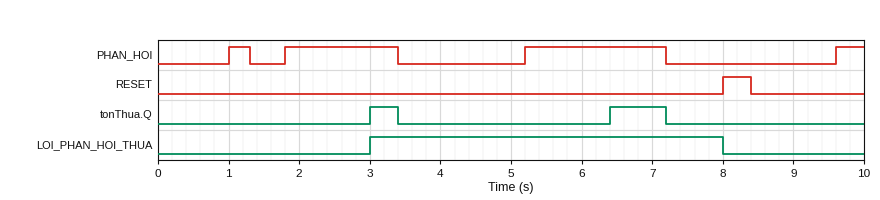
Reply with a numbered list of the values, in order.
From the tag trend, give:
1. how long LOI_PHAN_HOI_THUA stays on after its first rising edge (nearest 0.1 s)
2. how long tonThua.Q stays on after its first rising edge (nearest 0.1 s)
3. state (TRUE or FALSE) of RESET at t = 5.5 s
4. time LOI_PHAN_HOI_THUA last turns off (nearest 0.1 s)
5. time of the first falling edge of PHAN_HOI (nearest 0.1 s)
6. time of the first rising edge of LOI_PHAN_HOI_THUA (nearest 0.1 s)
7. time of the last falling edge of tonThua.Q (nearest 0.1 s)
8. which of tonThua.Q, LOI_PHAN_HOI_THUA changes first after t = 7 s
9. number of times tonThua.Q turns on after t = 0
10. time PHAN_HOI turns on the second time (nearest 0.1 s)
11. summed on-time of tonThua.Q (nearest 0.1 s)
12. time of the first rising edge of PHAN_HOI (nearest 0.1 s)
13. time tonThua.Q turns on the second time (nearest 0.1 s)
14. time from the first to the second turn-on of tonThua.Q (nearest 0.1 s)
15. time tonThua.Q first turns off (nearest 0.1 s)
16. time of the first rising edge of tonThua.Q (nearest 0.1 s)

1. 5.0 s
2. 0.4 s
3. FALSE
4. 8.0 s
5. 1.3 s
6. 3.0 s
7. 7.2 s
8. tonThua.Q
9. 2
10. 1.8 s
11. 1.2 s
12. 1.0 s
13. 6.4 s
14. 3.4 s
15. 3.4 s
16. 3.0 s
